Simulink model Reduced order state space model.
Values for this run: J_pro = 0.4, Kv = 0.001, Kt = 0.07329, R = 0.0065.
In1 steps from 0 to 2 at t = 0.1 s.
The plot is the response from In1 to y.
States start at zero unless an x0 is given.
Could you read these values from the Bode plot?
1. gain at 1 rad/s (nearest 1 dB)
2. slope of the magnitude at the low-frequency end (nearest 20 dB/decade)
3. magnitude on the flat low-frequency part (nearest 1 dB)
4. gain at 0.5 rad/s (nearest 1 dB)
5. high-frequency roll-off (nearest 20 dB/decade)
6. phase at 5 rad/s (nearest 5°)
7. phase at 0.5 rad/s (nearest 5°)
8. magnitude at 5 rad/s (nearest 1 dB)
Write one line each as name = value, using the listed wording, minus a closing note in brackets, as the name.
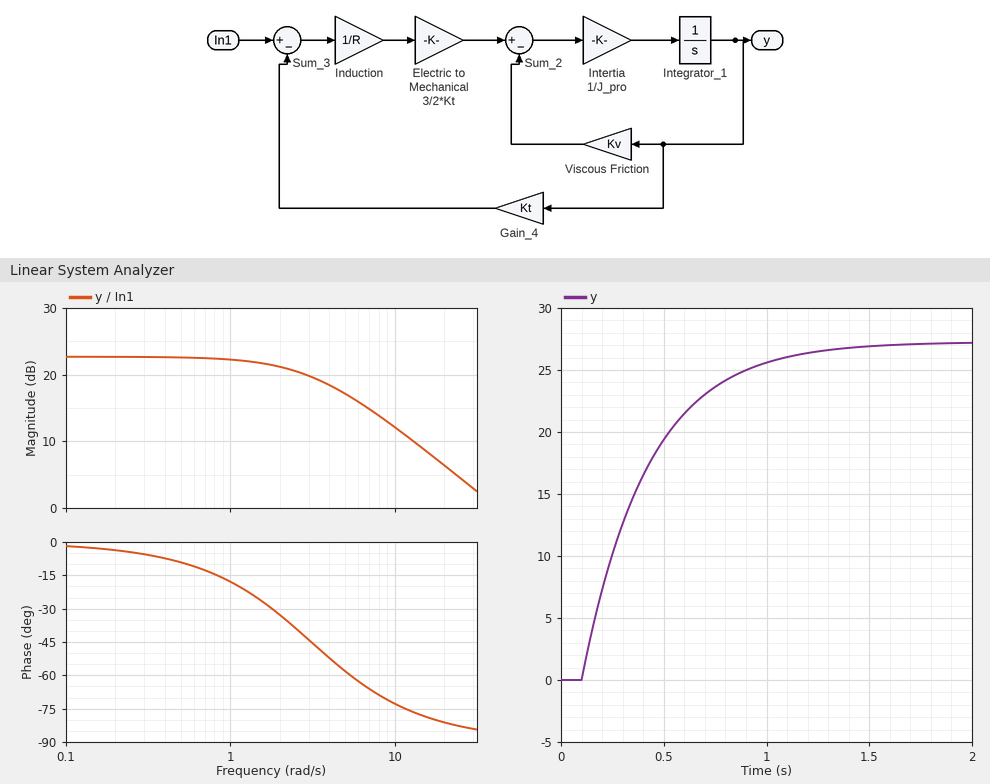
gain at 1 rad/s = 22 dB
slope of the magnitude at the low-frequency end = 0 dB/decade
magnitude on the flat low-frequency part = 23 dB
gain at 0.5 rad/s = 23 dB
high-frequency roll-off = -20 dB/decade
phase at 5 rad/s = -60°
phase at 0.5 rad/s = -10°
magnitude at 5 rad/s = 17 dB
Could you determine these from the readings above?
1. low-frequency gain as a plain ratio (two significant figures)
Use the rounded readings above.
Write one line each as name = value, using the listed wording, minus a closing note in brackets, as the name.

low-frequency gain as a plain ratio = 14
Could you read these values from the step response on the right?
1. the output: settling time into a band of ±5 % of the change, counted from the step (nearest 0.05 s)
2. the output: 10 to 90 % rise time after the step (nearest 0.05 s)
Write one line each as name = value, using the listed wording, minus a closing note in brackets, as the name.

the output: settling time into a band of ±5 % of the change, counted from the step = 0.95 s
the output: 10 to 90 % rise time after the step = 0.70 s
